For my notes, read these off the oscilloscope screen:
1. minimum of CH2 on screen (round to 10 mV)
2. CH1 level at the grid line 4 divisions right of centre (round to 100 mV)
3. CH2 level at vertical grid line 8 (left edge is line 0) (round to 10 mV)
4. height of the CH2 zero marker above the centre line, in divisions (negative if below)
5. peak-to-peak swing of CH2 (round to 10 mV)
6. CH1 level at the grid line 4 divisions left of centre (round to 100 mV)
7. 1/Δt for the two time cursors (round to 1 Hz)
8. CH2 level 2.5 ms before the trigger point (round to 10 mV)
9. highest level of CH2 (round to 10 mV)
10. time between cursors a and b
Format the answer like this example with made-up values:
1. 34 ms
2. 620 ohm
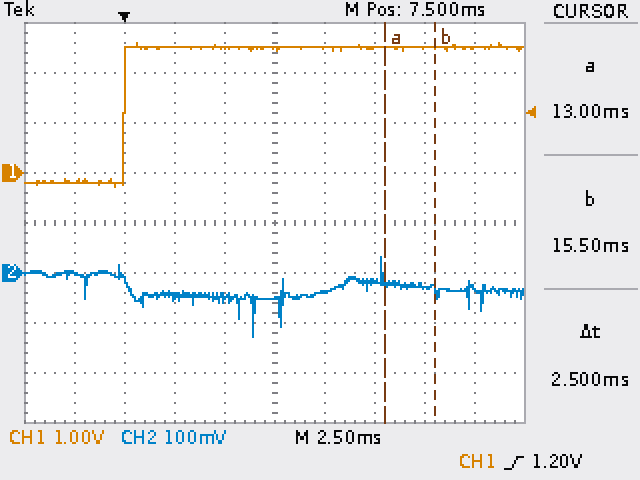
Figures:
1. -130 mV
2. 2.5 V
3. -30 mV
4. -1.0 div
5. 160 mV
6. -200 mV
7. 400 Hz
8. 0 mV
9. 30 mV
10. 2.5 ms
